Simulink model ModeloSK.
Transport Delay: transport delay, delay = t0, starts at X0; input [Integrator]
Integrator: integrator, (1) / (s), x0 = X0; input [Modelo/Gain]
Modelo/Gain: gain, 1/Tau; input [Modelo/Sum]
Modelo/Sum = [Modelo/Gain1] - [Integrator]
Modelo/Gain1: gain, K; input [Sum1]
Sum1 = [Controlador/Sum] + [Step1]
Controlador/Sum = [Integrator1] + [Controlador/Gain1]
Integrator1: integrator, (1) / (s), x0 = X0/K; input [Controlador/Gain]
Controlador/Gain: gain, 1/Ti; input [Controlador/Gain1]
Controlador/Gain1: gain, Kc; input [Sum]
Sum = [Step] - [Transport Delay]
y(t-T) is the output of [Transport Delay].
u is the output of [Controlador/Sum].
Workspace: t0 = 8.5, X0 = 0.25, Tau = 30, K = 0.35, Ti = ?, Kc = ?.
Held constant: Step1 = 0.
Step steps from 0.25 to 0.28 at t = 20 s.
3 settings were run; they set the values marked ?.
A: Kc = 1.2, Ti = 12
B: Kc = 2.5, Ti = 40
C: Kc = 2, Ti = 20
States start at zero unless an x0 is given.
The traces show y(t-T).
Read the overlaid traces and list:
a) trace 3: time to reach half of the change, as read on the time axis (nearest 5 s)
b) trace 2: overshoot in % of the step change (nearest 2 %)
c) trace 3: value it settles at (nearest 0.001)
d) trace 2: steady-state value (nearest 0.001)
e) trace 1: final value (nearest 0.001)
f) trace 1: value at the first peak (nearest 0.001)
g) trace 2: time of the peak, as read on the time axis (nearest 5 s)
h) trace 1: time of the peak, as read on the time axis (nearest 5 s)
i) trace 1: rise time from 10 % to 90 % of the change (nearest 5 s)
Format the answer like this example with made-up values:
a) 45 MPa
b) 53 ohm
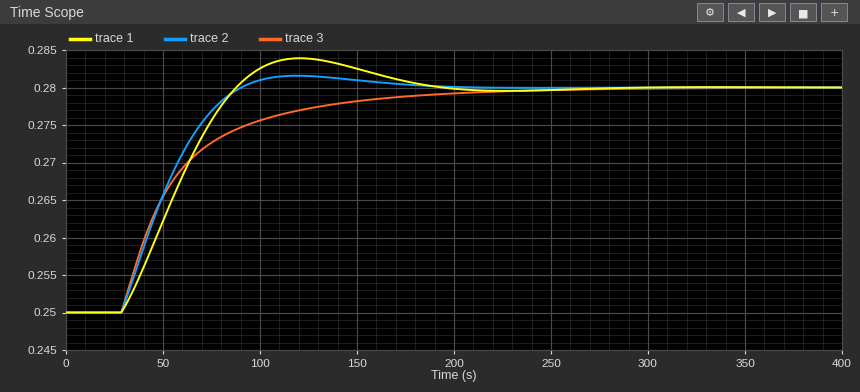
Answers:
a) 50 s
b) 6 %
c) 0.280
d) 0.280
e) 0.280
f) 0.284
g) 120 s
h) 120 s
i) 45 s
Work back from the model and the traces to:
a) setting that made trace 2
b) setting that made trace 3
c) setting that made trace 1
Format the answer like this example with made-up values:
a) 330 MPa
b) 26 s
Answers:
a) C
b) B
c) A
